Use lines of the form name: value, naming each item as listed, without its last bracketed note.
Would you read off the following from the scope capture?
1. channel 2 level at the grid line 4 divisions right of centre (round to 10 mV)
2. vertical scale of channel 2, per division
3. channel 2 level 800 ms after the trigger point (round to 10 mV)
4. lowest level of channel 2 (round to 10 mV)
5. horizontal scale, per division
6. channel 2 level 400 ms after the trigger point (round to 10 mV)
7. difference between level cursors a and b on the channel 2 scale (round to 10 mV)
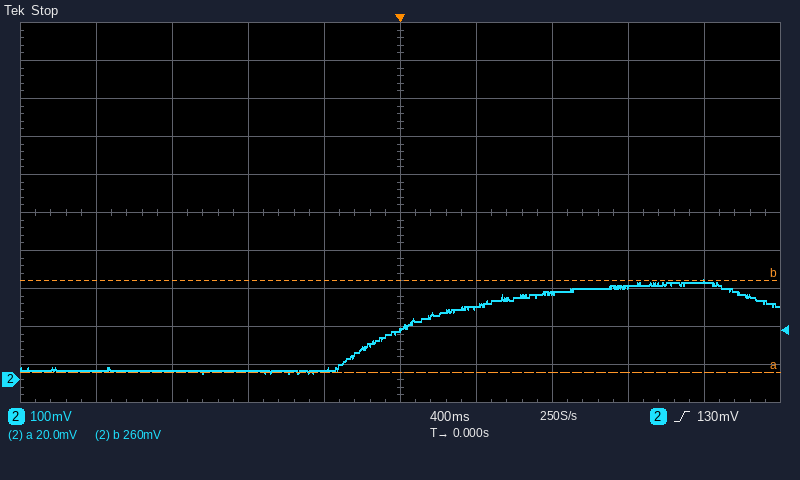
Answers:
channel 2 level at the grid line 4 divisions right of centre: 260 mV
vertical scale of channel 2, per division: 100 mV
channel 2 level 800 ms after the trigger point: 230 mV
lowest level of channel 2: 20 mV
horizontal scale, per division: 400 ms
channel 2 level 400 ms after the trigger point: 190 mV
difference between level cursors a and b on the channel 2 scale: 240 mV
